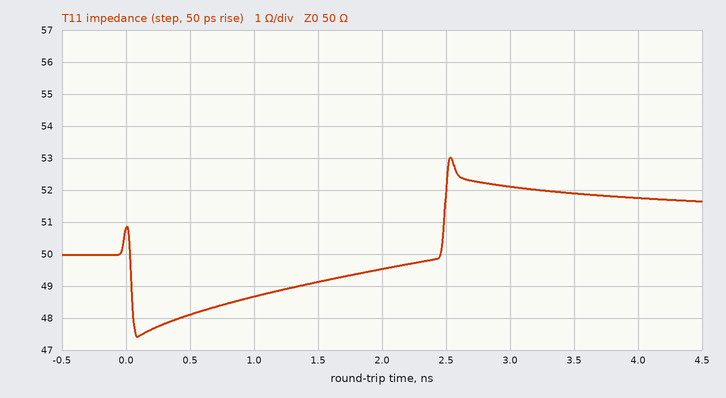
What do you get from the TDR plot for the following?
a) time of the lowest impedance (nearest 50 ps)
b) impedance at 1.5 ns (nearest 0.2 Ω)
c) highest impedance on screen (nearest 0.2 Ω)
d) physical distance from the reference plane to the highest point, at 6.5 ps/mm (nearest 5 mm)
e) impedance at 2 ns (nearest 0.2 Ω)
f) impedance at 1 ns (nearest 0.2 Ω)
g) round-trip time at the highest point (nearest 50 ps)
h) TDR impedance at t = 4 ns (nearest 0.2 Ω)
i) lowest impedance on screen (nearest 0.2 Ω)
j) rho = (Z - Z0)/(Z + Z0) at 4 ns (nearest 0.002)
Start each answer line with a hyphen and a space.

- 100 ps
- 49.2 Ω
- 53.0 Ω
- 195 mm
- 49.6 Ω
- 48.6 Ω
- 2.55 ns
- 51.8 Ω
- 47.4 Ω
- +0.018
